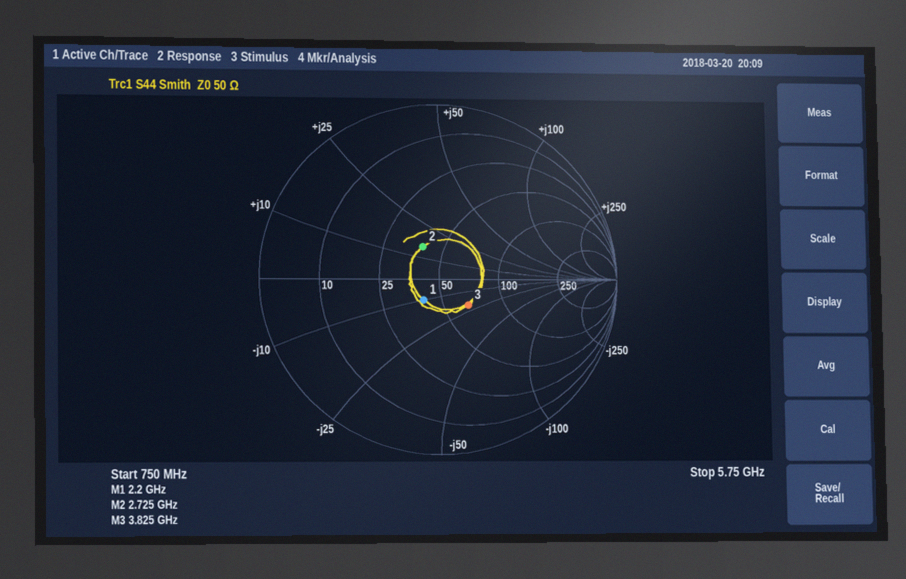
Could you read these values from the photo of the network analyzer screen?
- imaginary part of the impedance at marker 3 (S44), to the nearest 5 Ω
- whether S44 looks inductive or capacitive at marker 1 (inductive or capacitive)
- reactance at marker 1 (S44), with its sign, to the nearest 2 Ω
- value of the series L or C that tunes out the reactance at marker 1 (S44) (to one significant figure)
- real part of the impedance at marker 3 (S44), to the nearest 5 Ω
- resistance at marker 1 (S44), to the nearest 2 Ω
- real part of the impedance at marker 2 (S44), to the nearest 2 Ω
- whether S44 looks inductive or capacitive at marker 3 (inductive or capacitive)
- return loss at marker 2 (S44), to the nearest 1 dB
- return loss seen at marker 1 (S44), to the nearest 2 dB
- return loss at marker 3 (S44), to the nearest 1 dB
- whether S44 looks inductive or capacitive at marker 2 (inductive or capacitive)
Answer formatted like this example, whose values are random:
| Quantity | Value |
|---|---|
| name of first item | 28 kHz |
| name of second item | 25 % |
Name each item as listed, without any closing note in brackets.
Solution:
| Quantity | Value |
|---|---|
| imaginary part of the impedance at marker 3 (S44), to the nearest 5 Ω | -20 Ω |
| whether S44 looks inductive or capacitive at marker 1 | capacitive |
| reactance at marker 1 (S44), with its sign, to the nearest 2 Ω | -10 Ω |
| value of the series L or C that tunes out the reactance at marker 1 (S44) | 700 pH |
| real part of the impedance at marker 3 (S44), to the nearest 5 Ω | 65 Ω |
| resistance at marker 1 (S44), to the nearest 2 Ω | 40 Ω |
| real part of the impedance at marker 2 (S44), to the nearest 2 Ω | 40 Ω |
| whether S44 looks inductive or capacitive at marker 3 | capacitive |
| return loss at marker 2 (S44), to the nearest 1 dB | 14 dB |
| return loss seen at marker 1 (S44), to the nearest 2 dB | 16 dB |
| return loss at marker 3 (S44), to the nearest 1 dB | 13 dB |
| whether S44 looks inductive or capacitive at marker 2 | inductive |
